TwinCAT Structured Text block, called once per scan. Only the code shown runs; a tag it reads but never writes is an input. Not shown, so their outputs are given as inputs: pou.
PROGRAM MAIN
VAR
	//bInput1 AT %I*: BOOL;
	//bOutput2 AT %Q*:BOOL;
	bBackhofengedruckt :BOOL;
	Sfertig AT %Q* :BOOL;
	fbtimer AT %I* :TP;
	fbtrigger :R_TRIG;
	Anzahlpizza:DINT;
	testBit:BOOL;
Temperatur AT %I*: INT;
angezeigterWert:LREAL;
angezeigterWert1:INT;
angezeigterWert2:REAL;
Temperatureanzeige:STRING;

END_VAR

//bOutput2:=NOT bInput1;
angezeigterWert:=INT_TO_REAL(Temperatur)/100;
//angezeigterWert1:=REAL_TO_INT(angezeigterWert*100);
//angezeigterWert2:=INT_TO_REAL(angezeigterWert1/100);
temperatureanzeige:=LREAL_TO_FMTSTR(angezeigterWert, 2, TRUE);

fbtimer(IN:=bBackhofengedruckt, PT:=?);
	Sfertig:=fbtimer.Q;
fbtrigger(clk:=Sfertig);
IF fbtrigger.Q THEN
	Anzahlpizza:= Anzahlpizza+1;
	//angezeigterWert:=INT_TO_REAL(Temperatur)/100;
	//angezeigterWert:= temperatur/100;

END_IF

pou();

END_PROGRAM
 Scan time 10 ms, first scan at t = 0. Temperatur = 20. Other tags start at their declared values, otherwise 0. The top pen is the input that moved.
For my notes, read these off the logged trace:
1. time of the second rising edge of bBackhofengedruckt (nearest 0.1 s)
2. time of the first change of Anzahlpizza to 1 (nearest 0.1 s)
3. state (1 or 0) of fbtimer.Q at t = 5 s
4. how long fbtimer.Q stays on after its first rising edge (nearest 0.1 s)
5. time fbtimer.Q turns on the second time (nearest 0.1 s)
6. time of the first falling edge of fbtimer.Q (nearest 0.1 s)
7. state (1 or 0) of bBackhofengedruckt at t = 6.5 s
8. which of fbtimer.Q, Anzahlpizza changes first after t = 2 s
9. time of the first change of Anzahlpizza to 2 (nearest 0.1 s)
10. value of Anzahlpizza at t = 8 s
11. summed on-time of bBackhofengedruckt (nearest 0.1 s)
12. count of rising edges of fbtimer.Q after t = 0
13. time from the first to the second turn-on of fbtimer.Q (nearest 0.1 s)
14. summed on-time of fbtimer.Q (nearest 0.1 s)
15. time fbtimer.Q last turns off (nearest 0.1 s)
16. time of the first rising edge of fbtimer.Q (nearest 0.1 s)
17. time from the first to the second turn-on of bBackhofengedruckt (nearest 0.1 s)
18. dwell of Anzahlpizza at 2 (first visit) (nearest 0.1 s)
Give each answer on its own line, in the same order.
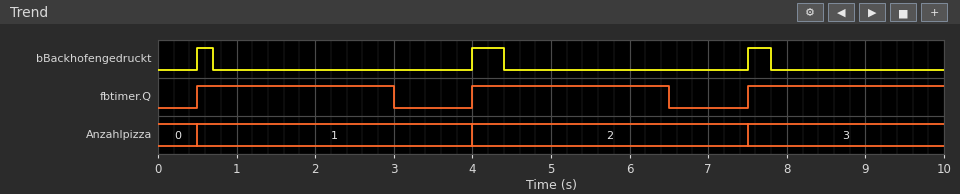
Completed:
4.0 s
0.5 s
1
2.5 s
4.0 s
3.0 s
0
fbtimer.Q
4.0 s
3
0.9 s
3
3.5 s
7.5 s
6.5 s
0.5 s
3.5 s
3.5 s
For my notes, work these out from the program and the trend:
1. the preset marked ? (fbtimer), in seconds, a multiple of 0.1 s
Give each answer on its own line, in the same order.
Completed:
2.5 s
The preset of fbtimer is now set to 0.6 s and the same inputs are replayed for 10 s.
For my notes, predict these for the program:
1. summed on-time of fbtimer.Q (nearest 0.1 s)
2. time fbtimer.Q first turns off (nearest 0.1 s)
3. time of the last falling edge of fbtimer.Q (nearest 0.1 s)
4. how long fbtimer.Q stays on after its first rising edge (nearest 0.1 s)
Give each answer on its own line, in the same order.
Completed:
1.8 s
1.1 s
8.1 s
0.6 s
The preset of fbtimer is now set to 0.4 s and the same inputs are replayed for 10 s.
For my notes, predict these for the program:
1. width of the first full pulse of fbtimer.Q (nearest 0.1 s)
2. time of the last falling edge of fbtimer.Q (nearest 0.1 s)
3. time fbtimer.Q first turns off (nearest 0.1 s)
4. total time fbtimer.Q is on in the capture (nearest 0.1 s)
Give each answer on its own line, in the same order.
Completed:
0.4 s
7.9 s
0.9 s
1.2 s
